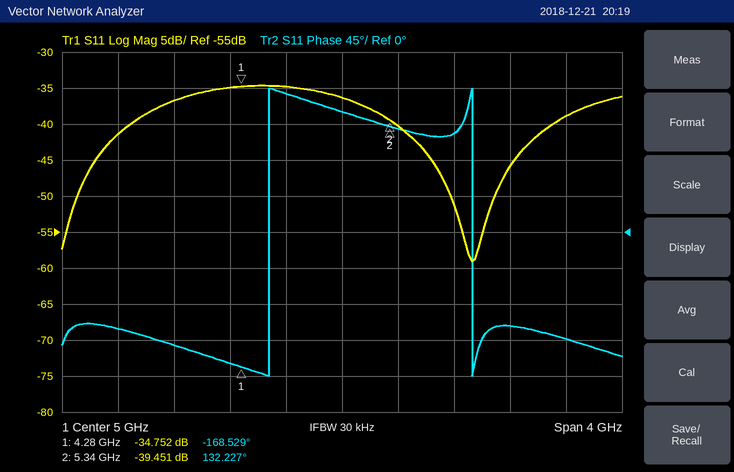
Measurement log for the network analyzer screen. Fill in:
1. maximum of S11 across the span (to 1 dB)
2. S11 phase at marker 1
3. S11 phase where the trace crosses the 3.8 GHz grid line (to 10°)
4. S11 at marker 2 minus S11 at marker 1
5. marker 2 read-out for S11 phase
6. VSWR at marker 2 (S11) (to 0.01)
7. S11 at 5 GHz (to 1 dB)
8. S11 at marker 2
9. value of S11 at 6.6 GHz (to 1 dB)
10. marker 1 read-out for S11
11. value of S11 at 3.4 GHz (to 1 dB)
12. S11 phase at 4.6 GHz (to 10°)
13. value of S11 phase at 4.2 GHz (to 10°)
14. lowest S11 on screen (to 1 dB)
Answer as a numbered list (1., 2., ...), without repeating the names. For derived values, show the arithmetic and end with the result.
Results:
1. -35 dB
2. -168.529°
3. -140°
4. -39.451 − (-34.752) = -4.699 dB
5. 132.227°
6. (1 + 0.0107)/(1 − 0.0107) ≈ 1.02
7. -36 dB
8. -39.451 dB
9. -39 dB
10. -34.752 dB
11. -41 dB
12. 170°
13. -160°
14. -59 dB
